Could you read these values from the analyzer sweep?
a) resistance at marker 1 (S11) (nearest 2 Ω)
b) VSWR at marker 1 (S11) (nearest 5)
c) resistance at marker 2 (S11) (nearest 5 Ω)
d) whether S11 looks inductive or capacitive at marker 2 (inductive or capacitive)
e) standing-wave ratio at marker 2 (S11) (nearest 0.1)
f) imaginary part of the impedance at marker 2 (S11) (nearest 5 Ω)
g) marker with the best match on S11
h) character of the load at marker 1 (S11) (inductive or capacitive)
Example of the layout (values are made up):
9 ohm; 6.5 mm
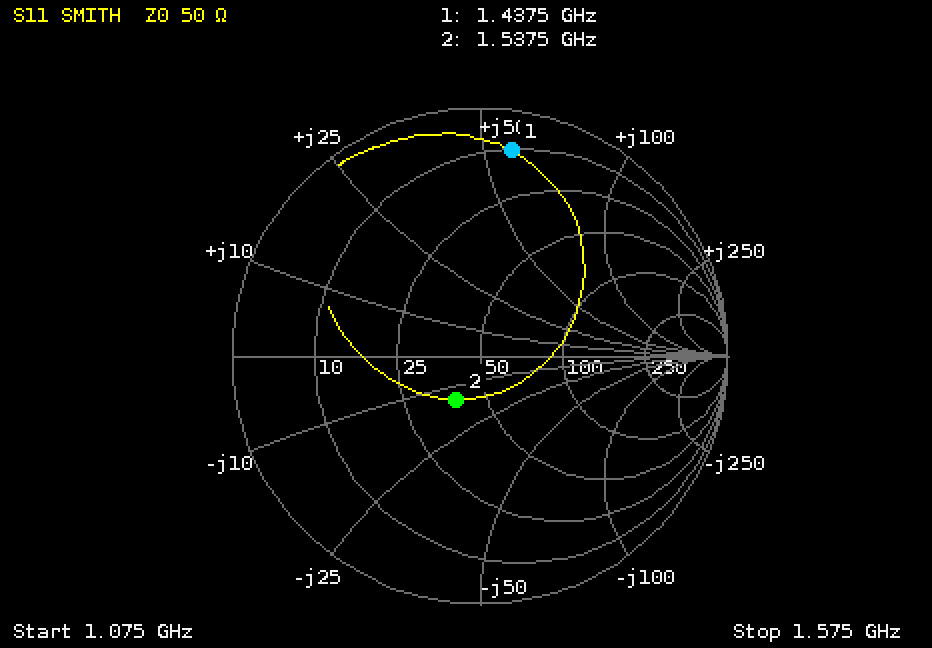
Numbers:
10 Ω; 10; 40 Ω; capacitive; 1.5; -15 Ω; marker 2; inductive
